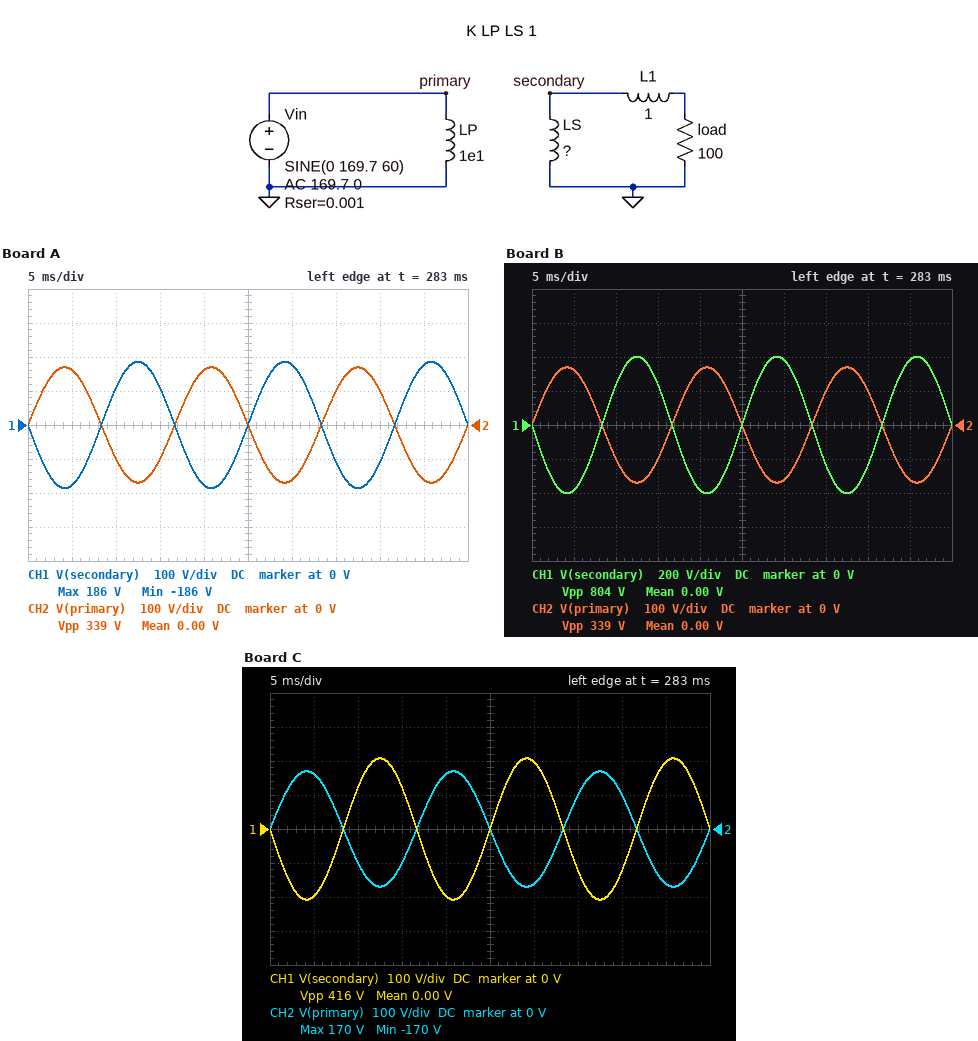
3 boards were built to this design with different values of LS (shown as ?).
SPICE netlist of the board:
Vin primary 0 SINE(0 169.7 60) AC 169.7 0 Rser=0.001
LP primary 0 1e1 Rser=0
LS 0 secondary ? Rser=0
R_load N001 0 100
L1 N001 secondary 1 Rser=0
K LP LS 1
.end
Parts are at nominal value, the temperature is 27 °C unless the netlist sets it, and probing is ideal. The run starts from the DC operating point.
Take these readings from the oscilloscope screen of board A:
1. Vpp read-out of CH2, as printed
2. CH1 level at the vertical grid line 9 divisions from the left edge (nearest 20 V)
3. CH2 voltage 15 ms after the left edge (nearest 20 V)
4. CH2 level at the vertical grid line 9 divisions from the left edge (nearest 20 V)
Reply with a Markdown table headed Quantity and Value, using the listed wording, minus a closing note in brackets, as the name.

| Quantity | Value |
|---|---|
| Vpp read-out of CH2, as printed | 339 V |
| CH1 level at the vertical grid line 9 divisions from the left edge | 180 V |
| CH2 voltage 15 ms after the left edge | -100 V |
| CH2 level at the vertical grid line 9 divisions from the left edge | -160 V |
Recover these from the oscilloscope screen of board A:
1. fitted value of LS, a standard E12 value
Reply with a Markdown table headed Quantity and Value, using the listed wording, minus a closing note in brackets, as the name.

| Quantity | Value |
|---|---|
| fitted value of LS, a standard E12 value | 12 H |
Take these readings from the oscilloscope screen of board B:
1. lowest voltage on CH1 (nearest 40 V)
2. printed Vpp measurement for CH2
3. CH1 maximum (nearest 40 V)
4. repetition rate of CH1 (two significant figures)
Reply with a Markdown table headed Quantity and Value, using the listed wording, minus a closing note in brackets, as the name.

| Quantity | Value |
|---|---|
| lowest voltage on CH1 | -400 V |
| printed Vpp measurement for CH2 | 339 V |
| CH1 maximum | 400 V |
| repetition rate of CH1 | 60 Hz |
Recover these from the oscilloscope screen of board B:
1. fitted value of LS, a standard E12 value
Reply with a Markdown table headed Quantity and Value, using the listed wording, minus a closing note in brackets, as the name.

| Quantity | Value |
|---|---|
| fitted value of LS, a standard E12 value | 56 H |
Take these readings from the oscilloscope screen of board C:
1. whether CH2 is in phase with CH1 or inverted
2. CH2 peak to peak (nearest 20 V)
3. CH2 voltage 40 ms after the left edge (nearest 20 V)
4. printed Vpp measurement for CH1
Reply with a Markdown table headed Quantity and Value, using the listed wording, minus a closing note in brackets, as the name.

| Quantity | Value |
|---|---|
| whether CH2 is in phase with CH1 or inverted | inverted |
| CH2 peak to peak | 340 V |
| CH2 voltage 40 ms after the left edge | 100 V |
| printed Vpp measurement for CH1 | 416 V |
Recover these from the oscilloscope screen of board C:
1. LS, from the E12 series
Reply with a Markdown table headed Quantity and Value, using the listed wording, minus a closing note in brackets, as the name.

| Quantity | Value |
|---|---|
| LS, from the E12 series | 15 H |
